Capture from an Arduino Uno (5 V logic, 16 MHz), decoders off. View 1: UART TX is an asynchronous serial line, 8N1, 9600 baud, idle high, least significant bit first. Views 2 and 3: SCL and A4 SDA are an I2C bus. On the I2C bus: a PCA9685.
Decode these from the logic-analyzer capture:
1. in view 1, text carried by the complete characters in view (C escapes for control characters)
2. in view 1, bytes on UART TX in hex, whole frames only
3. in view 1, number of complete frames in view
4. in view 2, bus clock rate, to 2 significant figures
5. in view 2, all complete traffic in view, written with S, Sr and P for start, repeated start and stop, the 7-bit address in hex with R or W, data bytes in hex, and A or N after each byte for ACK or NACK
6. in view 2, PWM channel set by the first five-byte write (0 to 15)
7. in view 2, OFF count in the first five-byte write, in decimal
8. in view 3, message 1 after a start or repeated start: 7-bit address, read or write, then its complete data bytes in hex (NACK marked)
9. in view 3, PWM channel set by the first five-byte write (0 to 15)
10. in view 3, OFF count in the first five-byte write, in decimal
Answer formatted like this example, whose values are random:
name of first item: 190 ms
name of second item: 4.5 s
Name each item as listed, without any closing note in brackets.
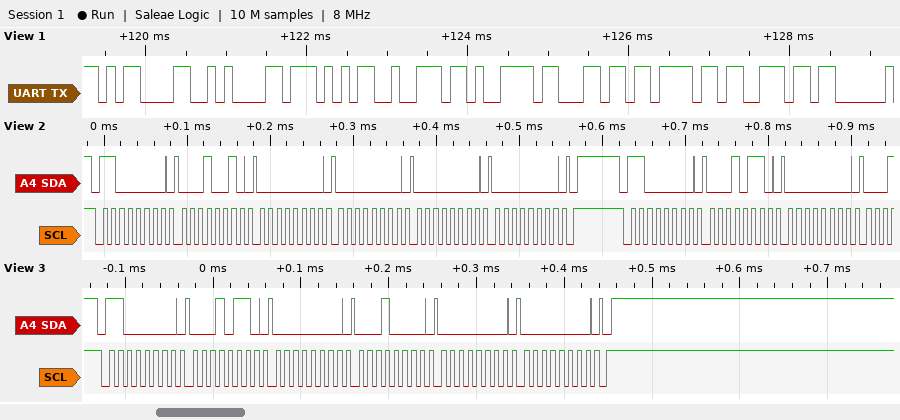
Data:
in view 1, text carried by the complete characters in view: "\r\nWrylon"
in view 1, bytes on UART TX in hex, whole frames only: 0D 0A 57 72 79 6C 6F 6E
in view 1, number of complete frames in view: 8
in view 2, bus clock rate, to 2 significant figures: 100 kHz
in view 2, all complete traffic in view, written with S, Sr and P for start, repeated start and stop, the 7-bit address in hex with R or W, data bytes in hex, and A or N after each byte for ACK or NACK: S 60W A 12 A 00 A 00 A 00 A 00 A P S 60W A 16 A 00 A
in view 2, PWM channel set by the first five-byte write: 3
in view 2, OFF count in the first five-byte write, in decimal: 0
in view 3, message 1 after a start or repeated start: 7-bit address, read or write, then its complete data bytes in hex: 0x60 write: 16 00 10 00 00
in view 3, PWM channel set by the first five-byte write: 4
in view 3, OFF count in the first five-byte write, in decimal: 0
